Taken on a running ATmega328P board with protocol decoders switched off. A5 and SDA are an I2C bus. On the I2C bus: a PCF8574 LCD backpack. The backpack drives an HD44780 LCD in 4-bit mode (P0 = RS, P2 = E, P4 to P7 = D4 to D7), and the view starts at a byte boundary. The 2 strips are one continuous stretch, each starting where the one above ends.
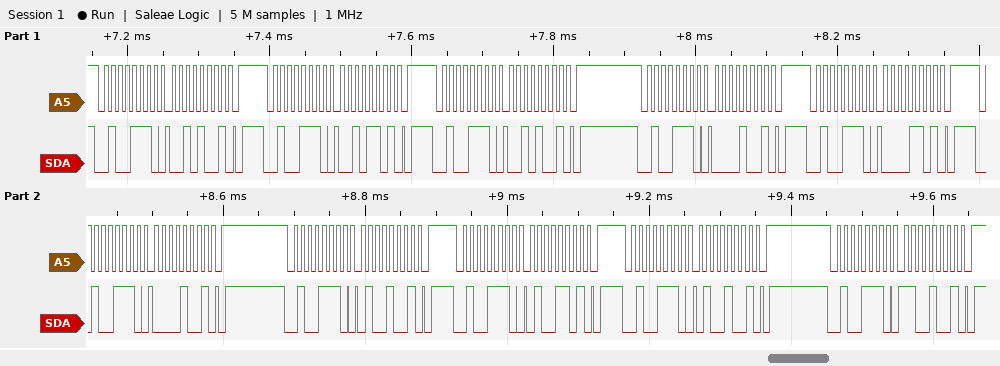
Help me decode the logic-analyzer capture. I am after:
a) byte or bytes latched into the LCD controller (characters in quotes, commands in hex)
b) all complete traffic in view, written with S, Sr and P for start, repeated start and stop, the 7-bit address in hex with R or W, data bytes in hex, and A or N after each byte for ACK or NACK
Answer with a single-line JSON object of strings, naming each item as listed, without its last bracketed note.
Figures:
{"byte or bytes latched into the LCD controller": "' '", "all complete traffic in view, written with S, Sr and P for start, repeated start and stop, the 7-bit address in hex with R or W, data bytes in hex, and A or N after each byte for ACK or NACK": "S 27W A 29 A P S 27W A 2D A P S 27W A 29 A P S 27W A 09 A P S 27W A 0D A P S 27W A 09 A P S 27W A 49 A P S 27W A 4D A P S 27W A 49 A P S 27W A C9 A P"}
